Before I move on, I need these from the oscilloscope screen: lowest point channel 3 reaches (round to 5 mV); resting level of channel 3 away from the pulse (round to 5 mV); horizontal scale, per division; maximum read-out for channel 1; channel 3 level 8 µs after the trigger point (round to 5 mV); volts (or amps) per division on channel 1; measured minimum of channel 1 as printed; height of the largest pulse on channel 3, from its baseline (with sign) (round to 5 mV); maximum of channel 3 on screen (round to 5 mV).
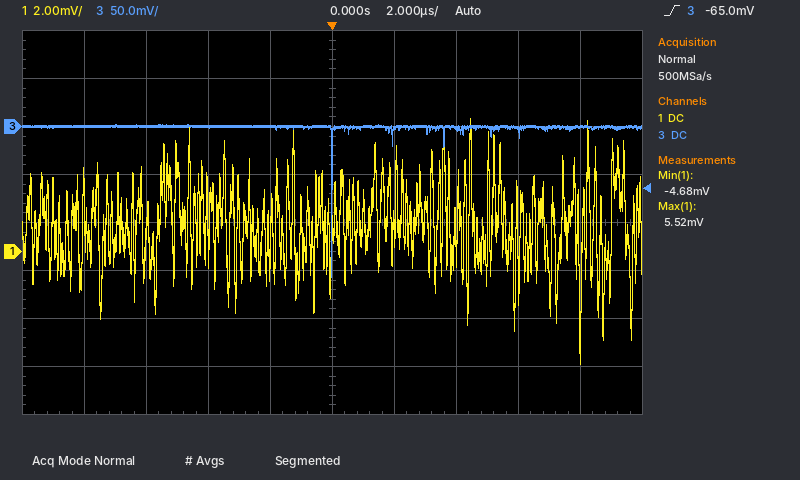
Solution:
-155 mV
0 mV
2 µs
5.52 mV
0 mV
2 mV
-4.68 mV
-155 mV
0 mV
